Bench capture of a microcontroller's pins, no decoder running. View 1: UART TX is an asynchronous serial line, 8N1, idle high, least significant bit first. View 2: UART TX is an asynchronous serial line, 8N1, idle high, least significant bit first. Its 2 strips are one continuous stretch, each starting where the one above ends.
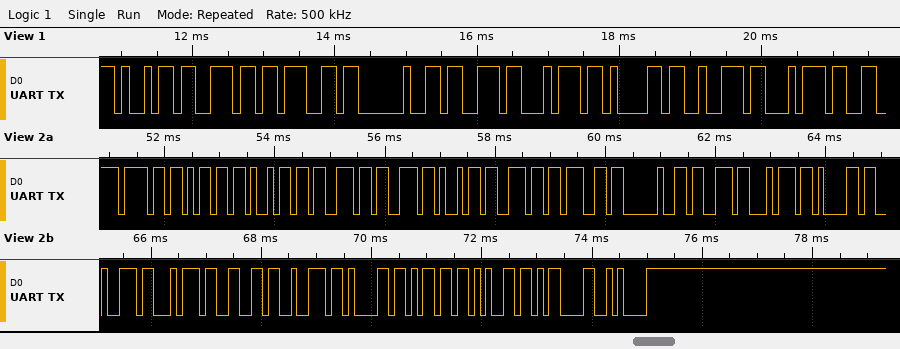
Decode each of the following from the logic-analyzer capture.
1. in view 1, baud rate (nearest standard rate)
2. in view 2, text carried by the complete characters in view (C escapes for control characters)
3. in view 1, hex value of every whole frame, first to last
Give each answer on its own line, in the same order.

9600 baud
"omissing startframe\r\n"
0x69 0x6E 0x67 0x20 0x73 0x74 0x61 0x72 0x74
